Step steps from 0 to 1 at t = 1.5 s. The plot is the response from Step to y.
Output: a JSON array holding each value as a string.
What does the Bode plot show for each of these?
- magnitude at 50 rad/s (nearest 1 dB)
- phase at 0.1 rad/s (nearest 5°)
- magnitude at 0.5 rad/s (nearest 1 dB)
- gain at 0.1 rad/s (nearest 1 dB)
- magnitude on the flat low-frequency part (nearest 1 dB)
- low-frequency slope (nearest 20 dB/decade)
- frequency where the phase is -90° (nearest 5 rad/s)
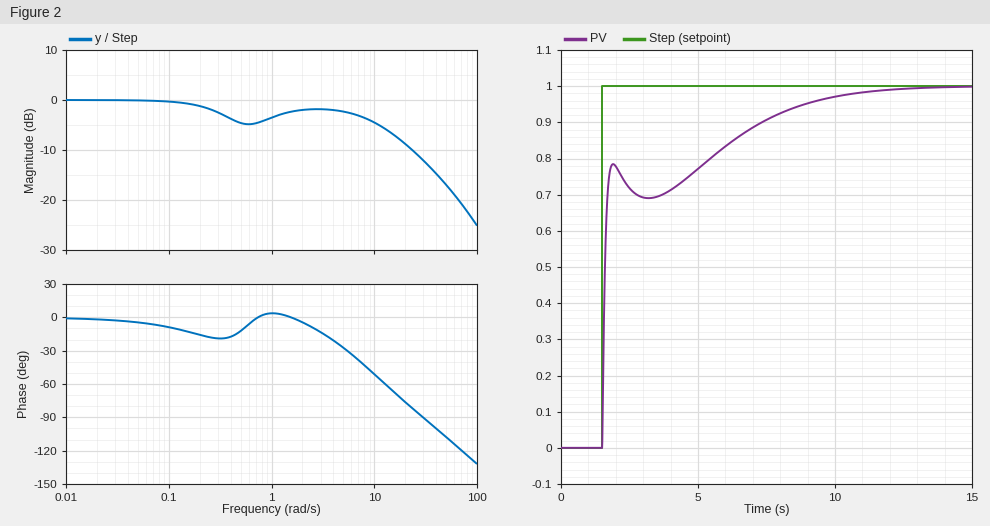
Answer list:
["-17 dB", "-10°", "-5 dB", "0 dB", "0 dB", "0 dB/decade", "30 rad/s"]
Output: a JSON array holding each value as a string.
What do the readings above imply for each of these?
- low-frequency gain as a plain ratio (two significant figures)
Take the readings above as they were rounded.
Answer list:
["1.0"]
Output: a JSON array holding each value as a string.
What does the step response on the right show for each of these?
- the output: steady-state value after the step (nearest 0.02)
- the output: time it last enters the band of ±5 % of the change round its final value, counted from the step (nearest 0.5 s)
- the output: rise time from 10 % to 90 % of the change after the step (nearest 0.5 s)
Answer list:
["1.00", "7.5 s", "6.0 s"]
